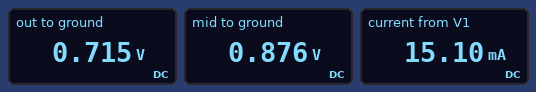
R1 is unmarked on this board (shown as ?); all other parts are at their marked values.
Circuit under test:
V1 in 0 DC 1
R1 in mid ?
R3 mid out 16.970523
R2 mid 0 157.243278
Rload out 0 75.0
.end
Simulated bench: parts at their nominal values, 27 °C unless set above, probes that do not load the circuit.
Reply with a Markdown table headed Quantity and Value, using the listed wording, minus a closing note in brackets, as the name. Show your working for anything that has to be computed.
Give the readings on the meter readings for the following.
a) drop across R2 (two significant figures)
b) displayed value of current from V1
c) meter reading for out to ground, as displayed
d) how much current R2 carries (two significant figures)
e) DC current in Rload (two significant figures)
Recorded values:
| Quantity | Value |
|---|---|
| drop across R2 | 876 mV = 880 mV |
| displayed value of current from V1 | 15.10 mA |
| meter reading for out to ground, as displayed | 0.715 V |
| how much current R2 carries | (876 mV) / 157.2 Ω = 5.6 mA |
| DC current in Rload | (715 mV) / 75 Ω = 9.5 mA |
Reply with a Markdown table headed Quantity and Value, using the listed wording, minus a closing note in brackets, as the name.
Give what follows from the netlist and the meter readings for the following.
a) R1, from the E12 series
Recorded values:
| Quantity | Value |
|---|---|
| R1, from the E12 series | 8.2 Ω |
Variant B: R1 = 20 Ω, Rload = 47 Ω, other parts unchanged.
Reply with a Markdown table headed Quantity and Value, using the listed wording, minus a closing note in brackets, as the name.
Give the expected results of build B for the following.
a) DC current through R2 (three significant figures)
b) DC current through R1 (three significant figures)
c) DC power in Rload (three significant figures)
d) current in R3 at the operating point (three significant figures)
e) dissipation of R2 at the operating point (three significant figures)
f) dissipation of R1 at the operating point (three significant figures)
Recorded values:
| Quantity | Value |
|---|---|
| DC current through R2 | 4.42 mA |
| DC current through R1 | 15.3 mA |
| DC power in Rload | 5.54 mW |
| current in R3 at the operating point | 10.9 mA |
| dissipation of R2 at the operating point | 3.07 mW |
| dissipation of R1 at the operating point | 4.67 mW |
